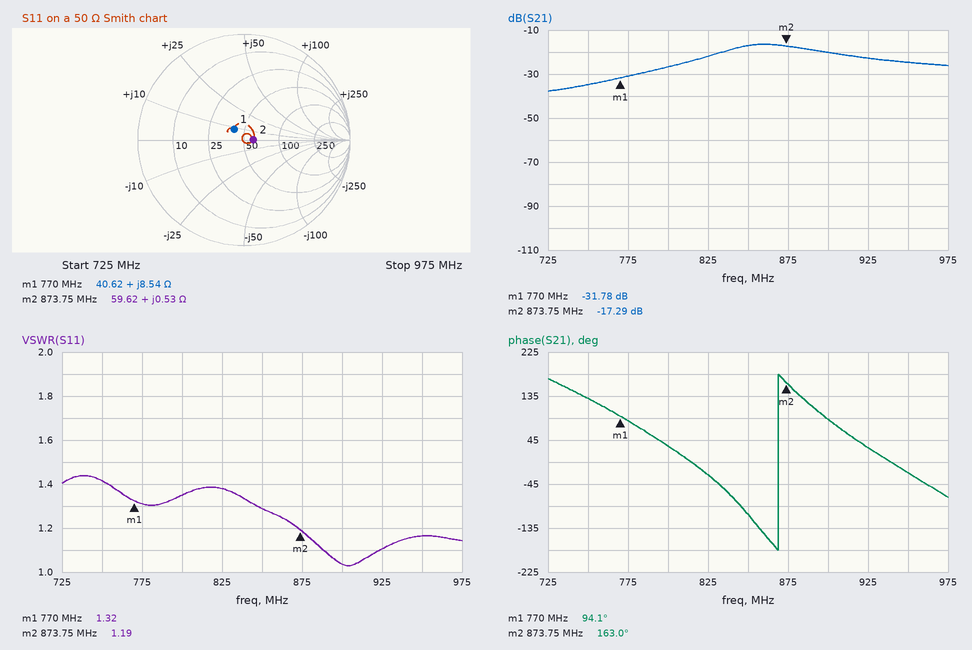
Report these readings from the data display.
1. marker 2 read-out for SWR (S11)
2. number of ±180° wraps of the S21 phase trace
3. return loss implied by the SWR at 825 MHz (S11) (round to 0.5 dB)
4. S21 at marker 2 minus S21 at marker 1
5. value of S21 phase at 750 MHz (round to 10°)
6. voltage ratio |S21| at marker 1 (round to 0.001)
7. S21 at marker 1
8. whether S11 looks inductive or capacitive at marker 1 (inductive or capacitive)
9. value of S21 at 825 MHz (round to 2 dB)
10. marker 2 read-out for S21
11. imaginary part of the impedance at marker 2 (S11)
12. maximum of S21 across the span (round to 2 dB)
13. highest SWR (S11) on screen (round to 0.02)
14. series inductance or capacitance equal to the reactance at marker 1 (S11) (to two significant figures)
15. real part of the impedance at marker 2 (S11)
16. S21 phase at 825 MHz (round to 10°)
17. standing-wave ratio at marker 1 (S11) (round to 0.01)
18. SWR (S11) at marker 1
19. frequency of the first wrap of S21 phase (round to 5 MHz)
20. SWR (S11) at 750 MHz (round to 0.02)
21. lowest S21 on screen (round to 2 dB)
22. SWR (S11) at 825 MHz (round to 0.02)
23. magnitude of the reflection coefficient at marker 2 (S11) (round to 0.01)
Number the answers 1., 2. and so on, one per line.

1. 1.19
2. 1
3. 16.0 dB
4. 14.49 dB
5. 130°
6. 0.026
7. -31.78 dB
8. inductive
9. -22 dB
10. -17.29 dB
11. +0.53 Ω
12. -16 dB
13. 1.44
14. 1.8 nH
15. 59.62 Ω
16. -30°
17. 1.32
18. 1.32
19. 870 MHz
20. 1.42
21. -38 dB
22. 1.38
23. 0.09
